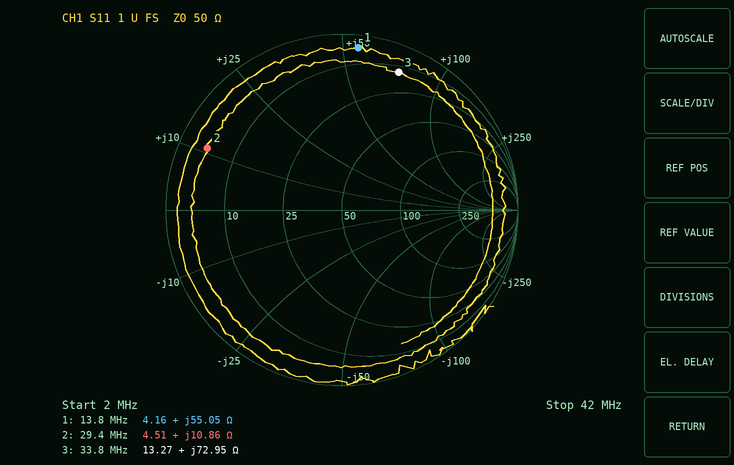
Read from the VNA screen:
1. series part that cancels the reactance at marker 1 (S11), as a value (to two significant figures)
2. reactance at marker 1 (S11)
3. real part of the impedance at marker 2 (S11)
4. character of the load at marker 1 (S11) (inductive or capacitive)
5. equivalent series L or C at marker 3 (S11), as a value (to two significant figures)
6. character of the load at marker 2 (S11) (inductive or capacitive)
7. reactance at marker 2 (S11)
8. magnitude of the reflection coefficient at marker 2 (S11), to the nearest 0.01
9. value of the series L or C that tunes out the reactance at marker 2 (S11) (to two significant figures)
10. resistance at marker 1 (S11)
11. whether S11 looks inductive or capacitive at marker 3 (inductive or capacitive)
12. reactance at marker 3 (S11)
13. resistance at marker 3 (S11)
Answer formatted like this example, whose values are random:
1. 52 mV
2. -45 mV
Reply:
1. 210 pF
2. +55.05 Ω
3. 4.51 Ω
4. inductive
5. 340 nH
6. inductive
7. +10.86 Ω
8. 0.84
9. 500 pF
10. 4.16 Ω
11. inductive
12. +72.95 Ω
13. 13.27 Ω
